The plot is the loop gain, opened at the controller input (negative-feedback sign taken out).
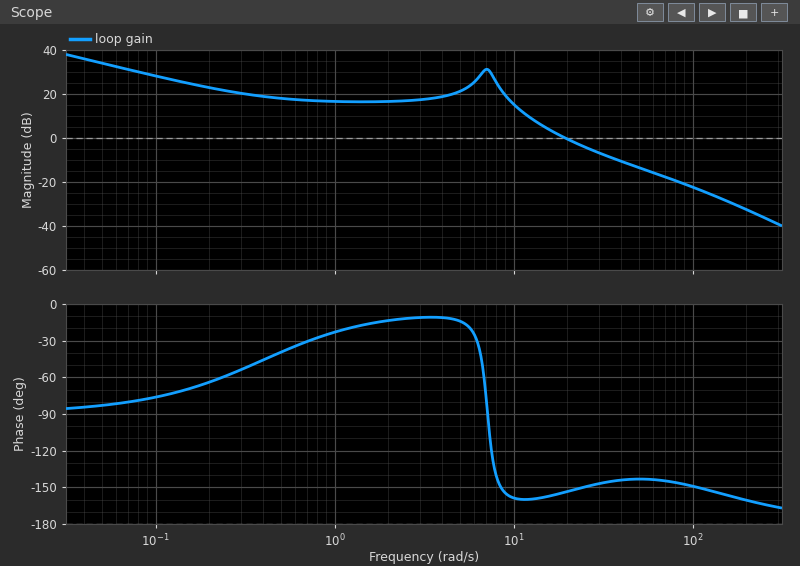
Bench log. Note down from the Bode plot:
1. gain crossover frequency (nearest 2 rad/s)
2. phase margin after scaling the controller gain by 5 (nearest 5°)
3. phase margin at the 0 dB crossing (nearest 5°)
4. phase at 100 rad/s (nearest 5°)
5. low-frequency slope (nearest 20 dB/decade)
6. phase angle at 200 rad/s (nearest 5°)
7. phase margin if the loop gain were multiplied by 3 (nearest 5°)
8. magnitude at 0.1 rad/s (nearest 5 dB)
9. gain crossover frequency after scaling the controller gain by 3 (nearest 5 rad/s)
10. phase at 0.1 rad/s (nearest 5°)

20 rad/s
35°
25°
-150°
-20 dB/decade
-160°
35°
30 dB
35 rad/s
-75°
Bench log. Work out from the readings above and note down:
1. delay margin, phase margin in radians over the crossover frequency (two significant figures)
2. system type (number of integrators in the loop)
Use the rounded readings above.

0.022 s
1
